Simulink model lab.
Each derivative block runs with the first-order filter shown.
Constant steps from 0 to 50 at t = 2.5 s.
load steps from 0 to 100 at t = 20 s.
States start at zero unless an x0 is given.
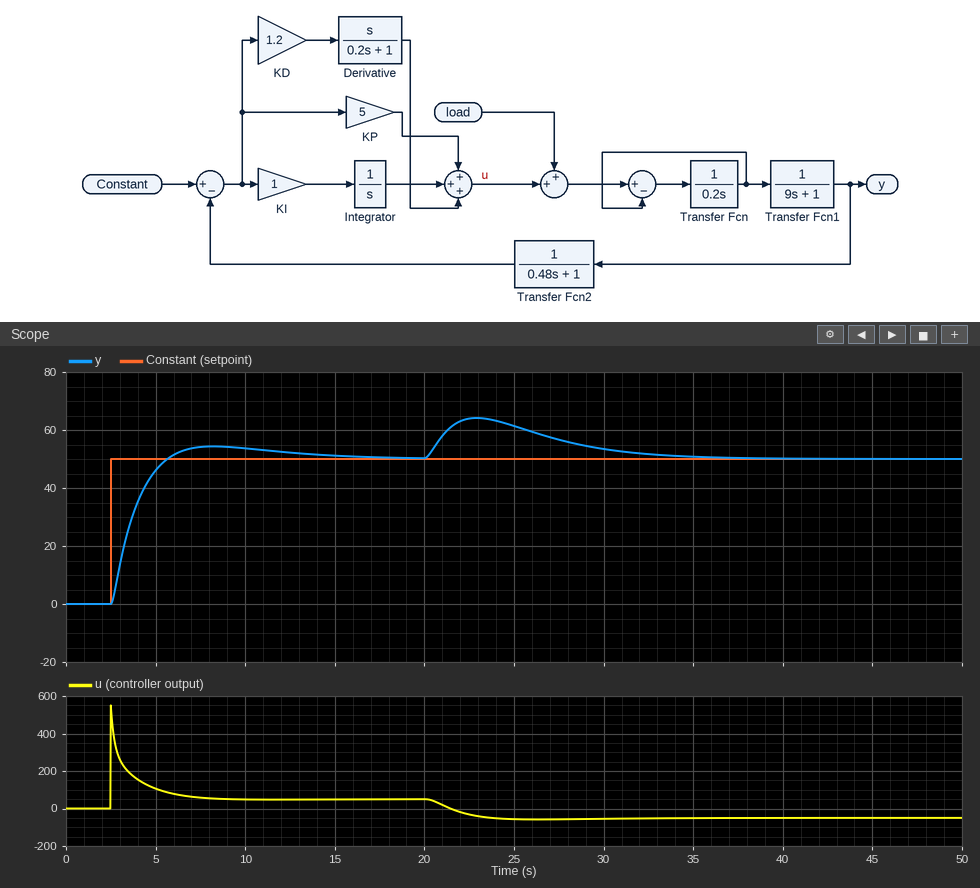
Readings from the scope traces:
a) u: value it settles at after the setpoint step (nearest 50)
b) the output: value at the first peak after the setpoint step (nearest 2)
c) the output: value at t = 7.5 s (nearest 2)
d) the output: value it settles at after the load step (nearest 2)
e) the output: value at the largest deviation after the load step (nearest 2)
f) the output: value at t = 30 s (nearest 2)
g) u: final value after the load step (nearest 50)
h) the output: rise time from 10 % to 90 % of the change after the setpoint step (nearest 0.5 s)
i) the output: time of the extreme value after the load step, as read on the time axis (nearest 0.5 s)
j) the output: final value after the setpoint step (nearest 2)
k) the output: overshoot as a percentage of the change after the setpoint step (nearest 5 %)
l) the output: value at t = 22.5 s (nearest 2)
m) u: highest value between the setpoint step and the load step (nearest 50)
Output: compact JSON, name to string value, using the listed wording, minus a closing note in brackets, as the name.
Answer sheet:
{"u: value it settles at after the setpoint step": "50", "the output: value at the first peak after the setpoint step": "54", "the output: value at t = 7.5 s": "54", "the output: value it settles at after the load step": "50", "the output: value at the largest deviation after the load step": "64", "the output: value at t = 30 s": "54", "u: final value after the load step": "-50", "the output: rise time from 10 % to 90 % of the change after the setpoint step": "2.0 s", "the output: time of the extreme value after the load step, as read on the time axis": "23.0 s", "the output: final value after the setpoint step": "50", "the output: overshoot as a percentage of the change after the setpoint step": "10 %", "the output: value at t = 22.5 s": "64", "u: highest value between the setpoint step and the load step": "550"}
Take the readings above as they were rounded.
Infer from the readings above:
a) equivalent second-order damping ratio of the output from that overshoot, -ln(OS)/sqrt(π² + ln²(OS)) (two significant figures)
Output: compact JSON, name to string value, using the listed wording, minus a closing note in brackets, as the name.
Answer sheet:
{"equivalent second-order damping ratio of the output from that overshoot, -ln(OS)/sqrt(π² + ln²(OS))": "0.59"}
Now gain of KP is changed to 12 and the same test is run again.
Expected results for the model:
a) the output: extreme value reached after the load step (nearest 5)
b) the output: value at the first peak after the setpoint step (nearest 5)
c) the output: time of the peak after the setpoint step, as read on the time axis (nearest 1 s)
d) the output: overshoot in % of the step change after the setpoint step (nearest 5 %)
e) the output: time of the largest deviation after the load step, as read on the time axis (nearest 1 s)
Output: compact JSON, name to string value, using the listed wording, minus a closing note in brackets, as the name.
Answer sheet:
{"the output: extreme value reached after the load step": "60", "the output: value at the first peak after the setpoint step": "60", "the output: time of the peak after the setpoint step, as read on the time axis": "4 s", "the output: overshoot in % of the step change after the setpoint step": "20 %", "the output: time of the largest deviation after the load step, as read on the time axis": "22 s"}
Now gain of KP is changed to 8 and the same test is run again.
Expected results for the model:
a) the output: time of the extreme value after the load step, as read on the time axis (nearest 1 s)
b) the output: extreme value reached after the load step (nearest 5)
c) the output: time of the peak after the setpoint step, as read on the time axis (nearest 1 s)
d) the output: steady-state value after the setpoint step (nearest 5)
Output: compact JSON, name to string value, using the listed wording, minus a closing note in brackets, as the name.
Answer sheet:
{"the output: time of the extreme value after the load step, as read on the time axis": "22 s", "the output: extreme value reached after the load step": "60", "the output: time of the peak after the setpoint step, as read on the time axis": "5 s", "the output: steady-state value after the setpoint step": "50"}
